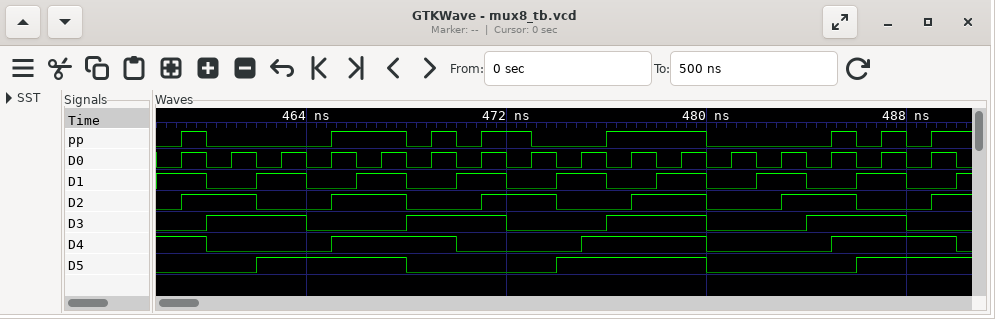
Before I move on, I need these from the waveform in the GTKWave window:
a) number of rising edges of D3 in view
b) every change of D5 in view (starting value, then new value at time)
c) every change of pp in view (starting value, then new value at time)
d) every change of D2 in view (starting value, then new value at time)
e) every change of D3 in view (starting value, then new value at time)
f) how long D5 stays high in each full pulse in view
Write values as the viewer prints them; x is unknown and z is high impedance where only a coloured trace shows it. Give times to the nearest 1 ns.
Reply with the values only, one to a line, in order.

4
0, 1 at 462 ns, 0 at 468 ns, 1 at 474 ns, 0 at 480 ns, 1 at 486 ns
0, 1 at 459 ns, 0 at 460 ns, 1 at 465 ns, 0 at 468 ns, 1 at 469 ns, 0 at 470 ns, 1 at 471 ns, 0 at 473 ns, 1 at 476 ns, 0 at 480 ns, 1 at 485 ns, 0 at 486 ns, 1 at 487 ns, 0 at 488 ns, 1 at 489 ns
0, 1 at 459 ns, 0 at 462 ns, 1 at 465 ns, 0 at 468 ns, 1 at 471 ns, 0 at 474 ns, 1 at 477 ns, 0 at 480 ns, 1 at 483 ns, 0 at 486 ns, 1 at 489 ns
0, 1 at 460 ns, 0 at 464 ns, 1 at 468 ns, 0 at 472 ns, 1 at 476 ns, 0 at 480 ns, 1 at 484 ns, 0 at 488 ns
6 ns, 6 ns
